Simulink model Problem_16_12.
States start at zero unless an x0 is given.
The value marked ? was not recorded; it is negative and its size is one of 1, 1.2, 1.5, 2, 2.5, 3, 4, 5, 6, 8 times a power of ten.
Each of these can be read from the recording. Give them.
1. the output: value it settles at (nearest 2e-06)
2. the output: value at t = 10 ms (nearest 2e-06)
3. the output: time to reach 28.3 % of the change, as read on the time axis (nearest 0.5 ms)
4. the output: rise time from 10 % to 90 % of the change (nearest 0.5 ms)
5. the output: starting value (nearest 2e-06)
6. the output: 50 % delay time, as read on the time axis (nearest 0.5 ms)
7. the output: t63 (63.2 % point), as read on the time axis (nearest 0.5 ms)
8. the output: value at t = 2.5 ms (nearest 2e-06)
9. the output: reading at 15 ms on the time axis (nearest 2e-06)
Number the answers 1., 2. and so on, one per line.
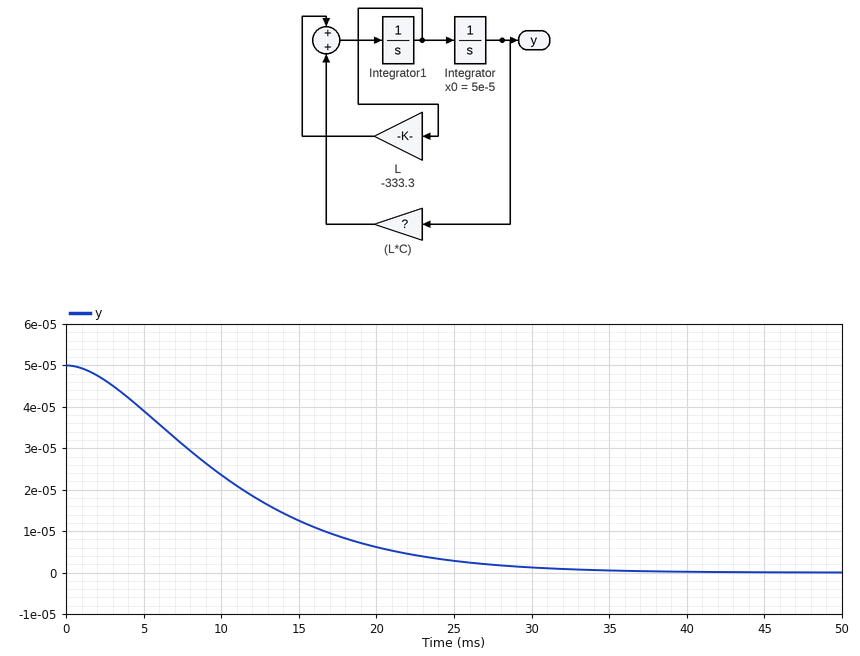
1. 0.000000
2. 0.000024
3. 6.0 ms
4. 18.5 ms
5. 0.000050
6. 9.5 ms
7. 12.0 ms
8. 0.000046
9. 0.000012
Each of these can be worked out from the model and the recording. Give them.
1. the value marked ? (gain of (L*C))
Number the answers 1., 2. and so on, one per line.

1. -30000
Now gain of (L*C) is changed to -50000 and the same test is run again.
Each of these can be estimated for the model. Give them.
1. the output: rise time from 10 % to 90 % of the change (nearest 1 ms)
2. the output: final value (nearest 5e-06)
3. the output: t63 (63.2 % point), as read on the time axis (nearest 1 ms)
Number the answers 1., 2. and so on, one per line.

1. 10 ms
2. 0.000000
3. 8 ms
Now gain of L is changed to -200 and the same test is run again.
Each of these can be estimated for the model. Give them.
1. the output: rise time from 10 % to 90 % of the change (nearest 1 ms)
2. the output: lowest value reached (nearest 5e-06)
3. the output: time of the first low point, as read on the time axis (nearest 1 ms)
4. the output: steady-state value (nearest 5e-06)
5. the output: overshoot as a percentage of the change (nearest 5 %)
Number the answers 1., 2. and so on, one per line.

1. 10 ms
2. -0.000005
3. 22 ms
4. 0.000000
5. 10 %
